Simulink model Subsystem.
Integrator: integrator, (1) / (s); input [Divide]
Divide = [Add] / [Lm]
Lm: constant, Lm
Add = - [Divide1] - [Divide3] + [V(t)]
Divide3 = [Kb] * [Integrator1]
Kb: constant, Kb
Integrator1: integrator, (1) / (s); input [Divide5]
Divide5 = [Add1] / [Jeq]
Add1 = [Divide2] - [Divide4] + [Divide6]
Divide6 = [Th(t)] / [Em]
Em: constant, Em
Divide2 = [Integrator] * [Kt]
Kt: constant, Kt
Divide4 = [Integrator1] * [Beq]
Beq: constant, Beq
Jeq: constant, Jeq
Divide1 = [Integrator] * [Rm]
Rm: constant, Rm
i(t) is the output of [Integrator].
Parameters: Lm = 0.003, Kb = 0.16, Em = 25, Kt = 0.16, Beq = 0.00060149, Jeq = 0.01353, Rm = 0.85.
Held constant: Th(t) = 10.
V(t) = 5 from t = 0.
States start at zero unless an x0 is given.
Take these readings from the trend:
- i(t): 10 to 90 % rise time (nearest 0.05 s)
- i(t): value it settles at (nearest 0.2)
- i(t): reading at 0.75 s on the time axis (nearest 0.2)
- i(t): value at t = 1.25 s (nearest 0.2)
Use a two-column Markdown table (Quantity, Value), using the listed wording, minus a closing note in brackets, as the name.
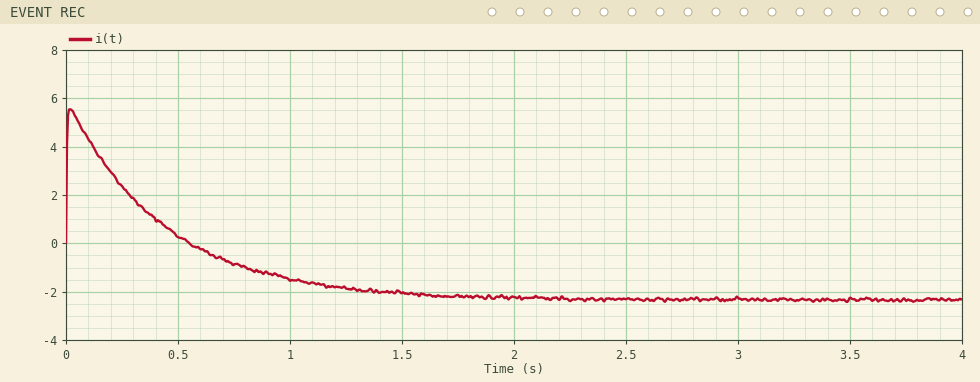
| Quantity | Value |
|---|---|
| i(t): 10 to 90 % rise time | 0.95 s |
| i(t): value it settles at | -2.4 |
| i(t): reading at 0.75 s on the time axis | -0.8 |
| i(t): value at t = 1.25 s | -1.8 |
